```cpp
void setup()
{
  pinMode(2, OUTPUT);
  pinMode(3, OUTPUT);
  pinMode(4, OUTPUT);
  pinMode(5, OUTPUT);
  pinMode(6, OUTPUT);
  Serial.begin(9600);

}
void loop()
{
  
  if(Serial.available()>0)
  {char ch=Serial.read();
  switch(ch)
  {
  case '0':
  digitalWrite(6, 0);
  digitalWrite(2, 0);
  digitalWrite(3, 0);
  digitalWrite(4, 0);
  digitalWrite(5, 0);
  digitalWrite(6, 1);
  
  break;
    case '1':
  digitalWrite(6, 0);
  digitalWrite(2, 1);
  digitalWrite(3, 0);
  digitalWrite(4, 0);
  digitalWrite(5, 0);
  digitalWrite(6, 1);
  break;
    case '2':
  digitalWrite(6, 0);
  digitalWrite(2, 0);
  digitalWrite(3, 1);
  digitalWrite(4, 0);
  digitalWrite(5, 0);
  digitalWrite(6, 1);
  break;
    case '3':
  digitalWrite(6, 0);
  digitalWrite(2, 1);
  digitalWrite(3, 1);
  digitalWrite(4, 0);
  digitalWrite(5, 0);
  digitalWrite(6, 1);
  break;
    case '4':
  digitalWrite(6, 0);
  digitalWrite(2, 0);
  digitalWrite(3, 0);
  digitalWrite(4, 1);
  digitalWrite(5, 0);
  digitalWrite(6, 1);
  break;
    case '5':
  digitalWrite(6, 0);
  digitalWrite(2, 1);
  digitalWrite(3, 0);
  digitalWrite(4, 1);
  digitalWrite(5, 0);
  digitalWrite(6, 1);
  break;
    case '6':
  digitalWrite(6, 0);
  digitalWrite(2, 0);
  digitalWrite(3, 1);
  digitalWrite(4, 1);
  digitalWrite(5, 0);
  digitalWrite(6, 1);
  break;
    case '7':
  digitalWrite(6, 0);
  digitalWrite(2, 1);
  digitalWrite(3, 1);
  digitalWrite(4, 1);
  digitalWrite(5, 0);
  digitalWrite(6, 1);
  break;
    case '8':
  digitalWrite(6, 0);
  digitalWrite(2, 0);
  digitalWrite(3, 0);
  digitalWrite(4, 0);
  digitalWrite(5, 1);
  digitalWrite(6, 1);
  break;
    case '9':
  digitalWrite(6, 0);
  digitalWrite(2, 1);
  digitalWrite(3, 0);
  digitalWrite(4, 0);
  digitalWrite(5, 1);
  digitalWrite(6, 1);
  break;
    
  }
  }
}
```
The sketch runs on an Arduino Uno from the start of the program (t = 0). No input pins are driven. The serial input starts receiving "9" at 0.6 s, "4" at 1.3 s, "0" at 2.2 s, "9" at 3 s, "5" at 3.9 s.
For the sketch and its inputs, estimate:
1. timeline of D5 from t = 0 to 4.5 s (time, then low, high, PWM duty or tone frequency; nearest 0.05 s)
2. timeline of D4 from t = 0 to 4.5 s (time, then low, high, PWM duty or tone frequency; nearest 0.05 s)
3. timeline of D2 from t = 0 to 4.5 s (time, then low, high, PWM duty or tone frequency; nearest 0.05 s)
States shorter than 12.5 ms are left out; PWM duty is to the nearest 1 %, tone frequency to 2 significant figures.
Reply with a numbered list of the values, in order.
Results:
1. 0 s low; 0.6 s high; 1.3 s low; 3 s high; 3.9 s low
2. 0 s low; 1.3 s high; 2.2 s low; 3.9 s high
3. 0 s low; 0.6 s high; 1.3 s low; 3 s high
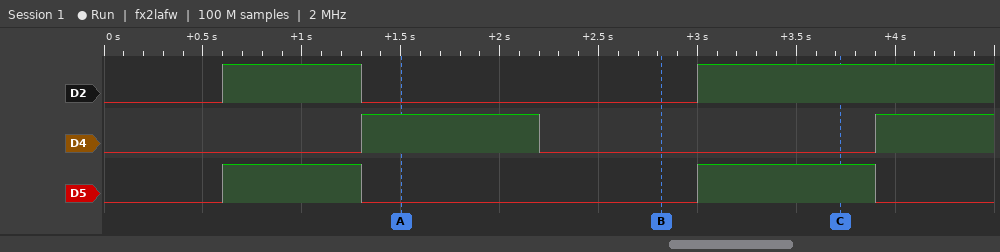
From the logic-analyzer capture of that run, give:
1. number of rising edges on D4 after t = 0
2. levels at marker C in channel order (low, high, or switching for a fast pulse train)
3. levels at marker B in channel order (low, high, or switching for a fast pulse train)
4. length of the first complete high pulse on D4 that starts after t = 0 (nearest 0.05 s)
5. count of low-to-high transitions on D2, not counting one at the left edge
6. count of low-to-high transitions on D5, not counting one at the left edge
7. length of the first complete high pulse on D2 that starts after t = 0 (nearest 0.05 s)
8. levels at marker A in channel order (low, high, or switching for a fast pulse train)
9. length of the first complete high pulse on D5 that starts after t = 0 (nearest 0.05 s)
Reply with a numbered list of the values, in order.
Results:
1. 2
2. D2 high, D4 low, D5 high
3. D2 low, D4 low, D5 low
4. 0.90 s
5. 2
6. 2
7. 0.70 s
8. D2 low, D4 high, D5 low
9. 0.70 s
